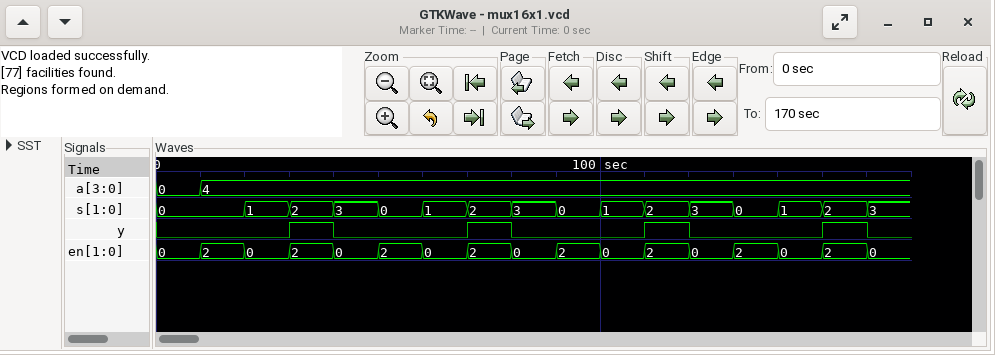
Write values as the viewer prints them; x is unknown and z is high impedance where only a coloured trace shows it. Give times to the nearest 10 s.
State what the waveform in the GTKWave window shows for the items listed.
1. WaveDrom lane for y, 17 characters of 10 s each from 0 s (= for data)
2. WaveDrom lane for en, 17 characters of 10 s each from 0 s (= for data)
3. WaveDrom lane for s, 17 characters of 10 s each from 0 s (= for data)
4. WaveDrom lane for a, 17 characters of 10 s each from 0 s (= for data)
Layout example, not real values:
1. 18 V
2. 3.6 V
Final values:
1. {name: 'y', wave: '0..10..10..10..10'}
2. {name: 'en', wave: '=================', data: '0 2 0 2 0 2 0 2 0 2 0 2 0 2 0 2 0'}
3. {name: 's', wave: '=.===============', data: '0 1 2 3 0 1 2 3 0 1 2 3 0 1 2 3'}
4. {name: 'a', wave: '==...............', data: '0 4'}
